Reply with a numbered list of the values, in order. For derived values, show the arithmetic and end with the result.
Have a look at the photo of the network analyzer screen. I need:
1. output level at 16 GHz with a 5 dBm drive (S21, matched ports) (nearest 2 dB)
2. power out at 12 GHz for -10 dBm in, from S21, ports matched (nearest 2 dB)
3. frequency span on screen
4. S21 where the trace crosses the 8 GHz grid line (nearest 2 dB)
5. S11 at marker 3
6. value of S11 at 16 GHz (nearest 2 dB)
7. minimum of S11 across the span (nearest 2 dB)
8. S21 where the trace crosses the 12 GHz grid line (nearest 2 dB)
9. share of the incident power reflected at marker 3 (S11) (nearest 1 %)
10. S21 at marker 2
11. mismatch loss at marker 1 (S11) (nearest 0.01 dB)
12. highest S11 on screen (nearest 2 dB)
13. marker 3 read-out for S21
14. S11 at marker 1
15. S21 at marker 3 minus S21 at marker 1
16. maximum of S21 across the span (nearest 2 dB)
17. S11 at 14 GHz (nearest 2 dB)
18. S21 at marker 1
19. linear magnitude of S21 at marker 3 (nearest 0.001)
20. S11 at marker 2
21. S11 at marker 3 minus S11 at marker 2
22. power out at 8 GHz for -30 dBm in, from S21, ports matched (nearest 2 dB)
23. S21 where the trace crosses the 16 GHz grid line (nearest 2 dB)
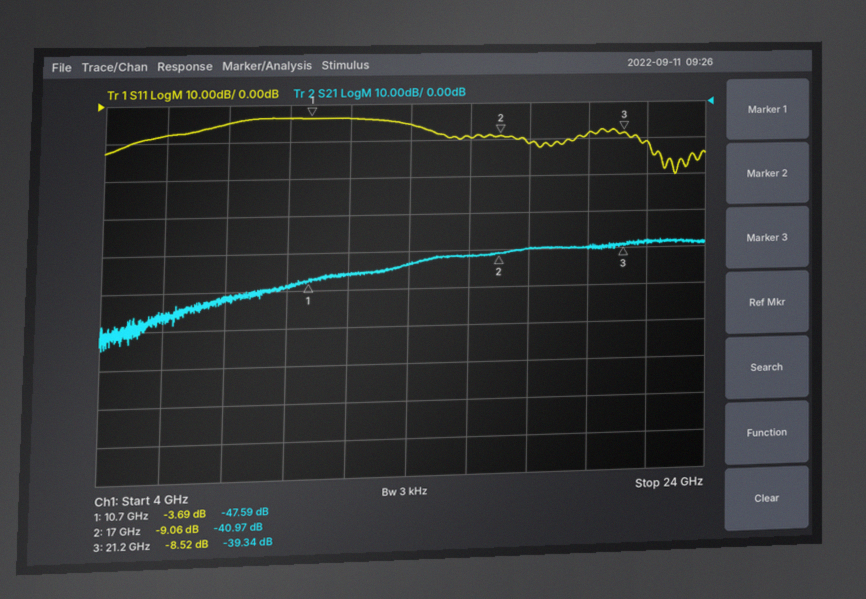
1. 5 dBm + (-42 dB) = -36 dBm
2. -10 dBm + (-46 dB) = -56 dBm
3. 20 GHz
4. -52 dB
5. -8.52 dB
6. -10 dB
7. -20 dB
8. -46 dB
9. 10^(-8.52/10) ≈ 14 %
10. -40.97 dB
11. −10 log10(1 − 10^(-3.69/10)) ≈ 2.42 dB
12. -4 dB
13. -39.34 dB
14. -3.69 dB
15. -39.34 − (-47.59) = 8.25 dB
16. -38 dB
17. -6 dB
18. -47.59 dB
19. 10^(-39.34/20) ≈ 0.011
20. -9.06 dB
21. -8.52 − (-9.06) = 0.54 dB
22. -30 dBm + (-52 dB) = -82 dBm
23. -42 dB
